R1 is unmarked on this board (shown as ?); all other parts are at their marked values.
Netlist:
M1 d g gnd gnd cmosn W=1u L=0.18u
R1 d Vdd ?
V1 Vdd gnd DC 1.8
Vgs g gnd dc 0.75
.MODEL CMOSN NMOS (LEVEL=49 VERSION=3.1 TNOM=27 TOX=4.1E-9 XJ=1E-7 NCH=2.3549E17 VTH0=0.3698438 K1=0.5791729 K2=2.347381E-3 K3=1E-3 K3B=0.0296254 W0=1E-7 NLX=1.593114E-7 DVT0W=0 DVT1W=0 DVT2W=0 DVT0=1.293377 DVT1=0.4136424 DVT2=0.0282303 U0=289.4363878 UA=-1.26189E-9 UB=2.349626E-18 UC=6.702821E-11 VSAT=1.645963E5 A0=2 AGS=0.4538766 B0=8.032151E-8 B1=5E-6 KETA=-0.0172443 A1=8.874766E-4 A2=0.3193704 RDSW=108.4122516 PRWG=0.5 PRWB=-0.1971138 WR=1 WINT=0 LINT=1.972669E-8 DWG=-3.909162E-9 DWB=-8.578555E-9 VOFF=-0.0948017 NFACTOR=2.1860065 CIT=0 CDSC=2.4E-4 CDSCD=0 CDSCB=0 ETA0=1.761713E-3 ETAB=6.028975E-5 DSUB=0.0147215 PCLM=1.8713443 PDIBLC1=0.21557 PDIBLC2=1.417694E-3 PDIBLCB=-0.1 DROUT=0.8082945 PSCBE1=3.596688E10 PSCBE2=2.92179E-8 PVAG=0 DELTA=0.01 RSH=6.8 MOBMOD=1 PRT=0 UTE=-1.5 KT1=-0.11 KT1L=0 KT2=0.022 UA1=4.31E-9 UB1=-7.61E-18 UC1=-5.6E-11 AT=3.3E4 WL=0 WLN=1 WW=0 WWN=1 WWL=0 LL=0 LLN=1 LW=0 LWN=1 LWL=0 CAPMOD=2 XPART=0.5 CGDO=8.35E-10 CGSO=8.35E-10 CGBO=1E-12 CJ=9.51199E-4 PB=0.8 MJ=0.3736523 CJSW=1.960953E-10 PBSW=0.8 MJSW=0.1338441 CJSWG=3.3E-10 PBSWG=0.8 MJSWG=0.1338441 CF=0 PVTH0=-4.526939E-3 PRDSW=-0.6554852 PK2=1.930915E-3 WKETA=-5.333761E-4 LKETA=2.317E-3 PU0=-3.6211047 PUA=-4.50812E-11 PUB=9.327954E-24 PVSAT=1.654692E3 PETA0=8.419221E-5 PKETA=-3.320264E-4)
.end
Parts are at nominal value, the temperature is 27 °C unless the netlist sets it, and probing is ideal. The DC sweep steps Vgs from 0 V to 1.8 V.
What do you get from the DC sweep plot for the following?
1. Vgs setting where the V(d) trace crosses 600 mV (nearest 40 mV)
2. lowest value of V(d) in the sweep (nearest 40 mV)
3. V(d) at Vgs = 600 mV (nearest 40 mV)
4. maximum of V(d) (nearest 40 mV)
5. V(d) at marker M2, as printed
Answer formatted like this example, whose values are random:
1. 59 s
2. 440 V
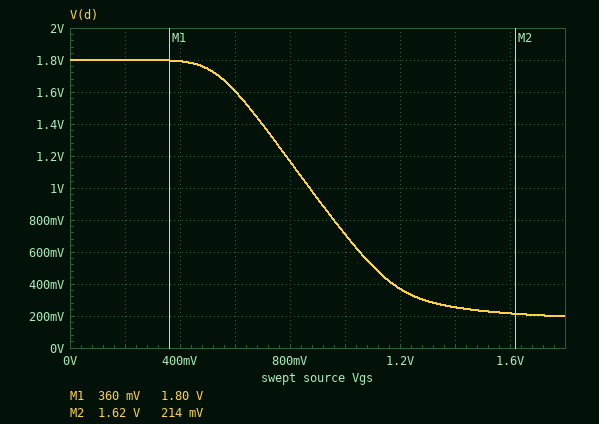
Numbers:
1. 1.04 V
2. 200 mV
3. 1.60 V
4. 1.80 V
5. 214 mV
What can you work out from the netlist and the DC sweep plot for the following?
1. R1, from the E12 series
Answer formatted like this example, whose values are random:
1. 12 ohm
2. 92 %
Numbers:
1. 5.6 kΩ
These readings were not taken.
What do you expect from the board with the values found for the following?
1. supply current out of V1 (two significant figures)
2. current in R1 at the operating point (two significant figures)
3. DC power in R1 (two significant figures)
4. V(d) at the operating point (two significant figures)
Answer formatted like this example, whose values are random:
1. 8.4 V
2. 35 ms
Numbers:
1. 92 µA
2. 92 µA
3. 48 µW
4. 1.3 V
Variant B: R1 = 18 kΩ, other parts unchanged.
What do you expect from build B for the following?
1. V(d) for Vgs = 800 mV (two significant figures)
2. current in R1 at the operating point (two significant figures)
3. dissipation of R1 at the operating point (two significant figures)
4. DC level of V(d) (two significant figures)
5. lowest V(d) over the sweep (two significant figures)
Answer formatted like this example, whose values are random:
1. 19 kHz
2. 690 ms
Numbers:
1. 260 mV
2. 76 µA
3. 100 µW
4. 430 mV
5. 60 mV
